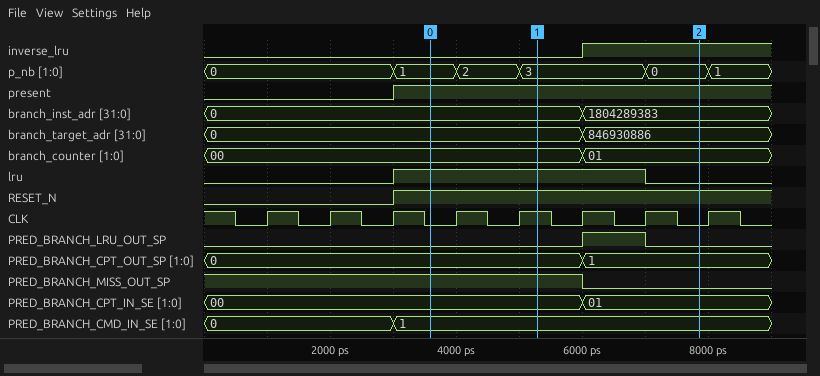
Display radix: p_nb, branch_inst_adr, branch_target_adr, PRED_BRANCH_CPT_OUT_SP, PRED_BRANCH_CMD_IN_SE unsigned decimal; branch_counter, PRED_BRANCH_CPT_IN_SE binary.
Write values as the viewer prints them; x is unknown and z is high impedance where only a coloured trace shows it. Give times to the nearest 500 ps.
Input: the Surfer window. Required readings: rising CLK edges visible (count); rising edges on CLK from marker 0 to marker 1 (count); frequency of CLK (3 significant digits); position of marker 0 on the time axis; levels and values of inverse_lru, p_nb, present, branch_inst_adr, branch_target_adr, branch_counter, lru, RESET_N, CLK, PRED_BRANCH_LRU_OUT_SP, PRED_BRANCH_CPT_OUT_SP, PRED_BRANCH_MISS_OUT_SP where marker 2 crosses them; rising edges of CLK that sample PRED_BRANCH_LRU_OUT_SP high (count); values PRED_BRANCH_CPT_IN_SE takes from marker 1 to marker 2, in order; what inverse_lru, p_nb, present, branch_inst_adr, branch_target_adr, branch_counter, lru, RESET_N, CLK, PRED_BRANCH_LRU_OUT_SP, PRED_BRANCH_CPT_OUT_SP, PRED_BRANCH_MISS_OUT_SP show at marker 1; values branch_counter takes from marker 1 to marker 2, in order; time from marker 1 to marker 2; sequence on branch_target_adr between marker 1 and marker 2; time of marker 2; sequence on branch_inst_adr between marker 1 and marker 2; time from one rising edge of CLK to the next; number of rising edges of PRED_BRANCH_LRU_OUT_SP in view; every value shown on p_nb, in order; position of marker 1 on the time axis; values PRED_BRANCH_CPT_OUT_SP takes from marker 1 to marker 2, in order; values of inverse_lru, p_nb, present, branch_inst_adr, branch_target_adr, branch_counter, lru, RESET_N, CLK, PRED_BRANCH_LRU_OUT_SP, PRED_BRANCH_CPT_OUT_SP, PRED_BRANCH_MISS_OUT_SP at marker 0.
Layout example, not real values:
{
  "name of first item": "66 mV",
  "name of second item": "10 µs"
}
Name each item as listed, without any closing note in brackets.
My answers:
{
  "rising CLK edges visible": "8",
  "rising edges on CLK from marker 0 to marker 1": "2",
  "frequency of CLK": "1.00 GHz",
  "position of marker 0 on the time axis": "3500 ps",
  "levels and values of inverse_lru, p_nb, present, branch_inst_adr, branch_target_adr, branch_counter, lru, RESET_N, CLK, PRED_BRANCH_LRU_OUT_SP, PRED_BRANCH_CPT_OUT_SP, PRED_BRANCH_MISS_OUT_SP where marker 2 crosses them": "inverse_lru=1, p_nb=0, present=1, branch_inst_adr=1804289383, branch_target_adr=846930886, branch_counter=01, lru=0, RESET_N=1, CLK=0, PRED_BRANCH_LRU_OUT_SP=0, PRED_BRANCH_CPT_OUT_SP=1, PRED_BRANCH_MISS_OUT_SP=0",
  "rising edges of CLK that sample PRED_BRANCH_LRU_OUT_SP high": "1",
  "values PRED_BRANCH_CPT_IN_SE takes from marker 1 to marker 2, in order": "00, 01",
  "what inverse_lru, p_nb, present, branch_inst_adr, branch_target_adr, branch_counter, lru, RESET_N, CLK, PRED_BRANCH_LRU_OUT_SP, PRED_BRANCH_CPT_OUT_SP, PRED_BRANCH_MISS_OUT_SP show at marker 1": "inverse_lru=0, p_nb=3, present=1, branch_inst_adr=0, branch_target_adr=0, branch_counter=00, lru=1, RESET_N=1, CLK=1, PRED_BRANCH_LRU_OUT_SP=0, PRED_BRANCH_CPT_OUT_SP=0, PRED_BRANCH_MISS_OUT_SP=1",
  "values branch_counter takes from marker 1 to marker 2, in order": "00, 01",
  "time from marker 1 to marker 2": "2500 ps",
  "sequence on branch_target_adr between marker 1 and marker 2": "0, 846930886",
  "time of marker 2": "8000 ps",
  "sequence on branch_inst_adr between marker 1 and marker 2": "0, 1804289383",
  "time from one rising edge of CLK to the next": "1000 ps",
  "number of rising edges of PRED_BRANCH_LRU_OUT_SP in view": "1",
  "every value shown on p_nb, in order": "0, 1, 2, 3, 0, 1",
  "position of marker 1 on the time axis": "5500 ps",
  "values PRED_BRANCH_CPT_OUT_SP takes from marker 1 to marker 2, in order": "0, 1",
  "values of inverse_lru, p_nb, present, branch_inst_adr, branch_target_adr, branch_counter, lru, RESET_N, CLK, PRED_BRANCH_LRU_OUT_SP, PRED_BRANCH_CPT_OUT_SP, PRED_BRANCH_MISS_OUT_SP at marker 0": "inverse_lru=0, p_nb=1, present=1, branch_inst_adr=0, branch_target_adr=0, branch_counter=00, lru=1, RESET_N=1, CLK=0, PRED_BRANCH_LRU_OUT_SP=0, PRED_BRANCH_CPT_OUT_SP=0, PRED_BRANCH_MISS_OUT_SP=1"
}
